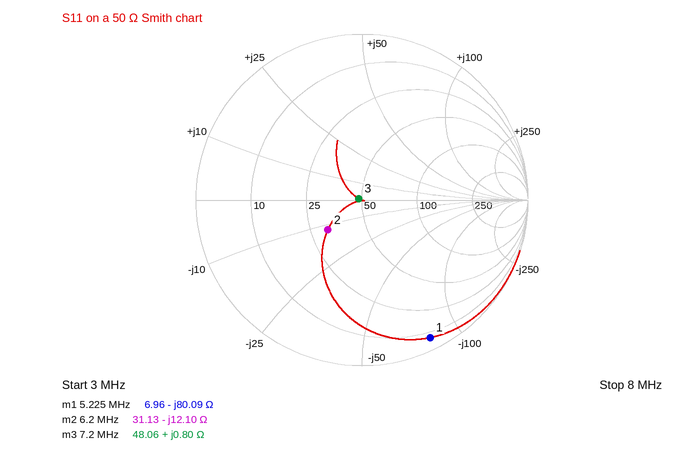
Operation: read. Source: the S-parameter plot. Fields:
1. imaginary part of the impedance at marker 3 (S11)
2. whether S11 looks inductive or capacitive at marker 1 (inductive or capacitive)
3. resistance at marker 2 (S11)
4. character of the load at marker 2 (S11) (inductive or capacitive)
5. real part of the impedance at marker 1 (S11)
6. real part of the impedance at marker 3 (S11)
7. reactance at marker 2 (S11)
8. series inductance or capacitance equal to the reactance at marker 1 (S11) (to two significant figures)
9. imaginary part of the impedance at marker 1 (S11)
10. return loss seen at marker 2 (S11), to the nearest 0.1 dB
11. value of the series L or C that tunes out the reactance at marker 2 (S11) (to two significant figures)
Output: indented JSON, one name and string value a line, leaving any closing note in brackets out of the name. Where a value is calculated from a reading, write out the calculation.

{
  "imaginary part of the impedance at marker 3": "+0.80 Ω",
  "whether S11 looks inductive or capacitive at marker 1": "capacitive",
  "resistance at marker 2": "31.13 Ω",
  "character of the load at marker 2 (S11)": "capacitive",
  "real part of the impedance at marker 1": "6.96 Ω",
  "real part of the impedance at marker 3": "48.06 Ω",
  "reactance at marker 2": "-12.10 Ω",
  "series inductance or capacitance equal to the reactance at marker 1 (S11)": "C = 1/(2π × 5.225 MHz × 80.09 Ω) ≈ 380 pF",
  "imaginary part of the impedance at marker 1": "-80.09 Ω",
  "return loss seen at marker 2 (S11), to the nearest 0.1 dB": "11.3 dB",
  "value of the series L or C that tunes out the reactance at marker 2 (S11)": "L = 12.1 Ω/(2π × 6.2 MHz) ≈ 311 nH, so 310 nH to two significant figures"
}
